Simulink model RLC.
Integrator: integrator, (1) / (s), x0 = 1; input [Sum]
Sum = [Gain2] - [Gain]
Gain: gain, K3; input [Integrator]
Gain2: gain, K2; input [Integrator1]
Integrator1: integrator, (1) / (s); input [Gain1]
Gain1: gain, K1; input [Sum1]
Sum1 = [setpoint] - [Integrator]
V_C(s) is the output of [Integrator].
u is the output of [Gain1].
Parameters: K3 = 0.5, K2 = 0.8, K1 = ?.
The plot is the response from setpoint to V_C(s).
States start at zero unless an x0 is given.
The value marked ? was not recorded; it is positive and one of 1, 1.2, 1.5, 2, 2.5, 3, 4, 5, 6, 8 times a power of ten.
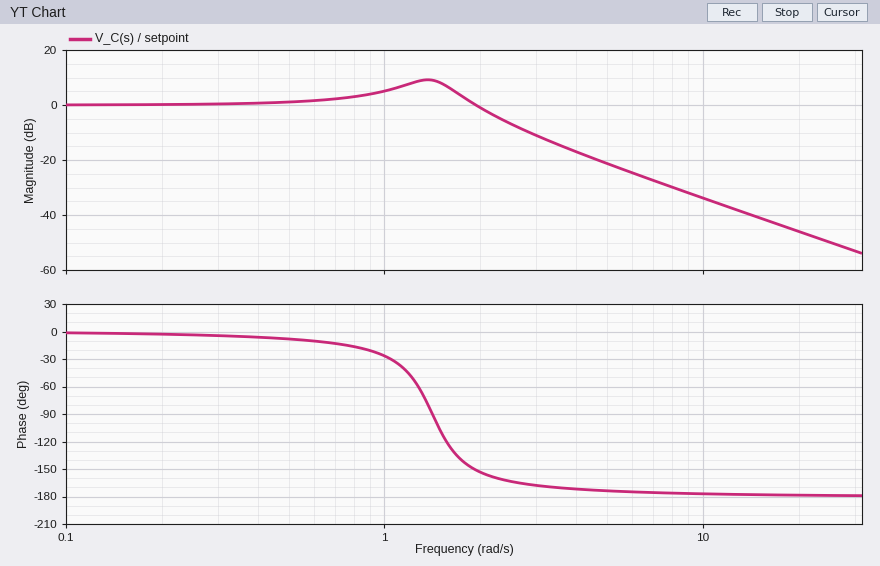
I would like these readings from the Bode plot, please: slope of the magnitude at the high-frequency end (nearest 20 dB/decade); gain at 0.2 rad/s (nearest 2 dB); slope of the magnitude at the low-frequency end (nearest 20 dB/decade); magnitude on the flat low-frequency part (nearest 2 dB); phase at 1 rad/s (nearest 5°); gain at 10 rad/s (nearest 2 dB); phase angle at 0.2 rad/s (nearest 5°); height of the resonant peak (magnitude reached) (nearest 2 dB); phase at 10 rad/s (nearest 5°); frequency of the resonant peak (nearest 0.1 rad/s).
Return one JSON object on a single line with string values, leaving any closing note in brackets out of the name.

{"slope of the magnitude at the high-frequency end": "-40 dB/decade", "gain at 0.2 rad/s": "0 dB", "slope of the magnitude at the low-frequency end": "0 dB/decade", "magnitude on the flat low-frequency part": "0 dB", "phase at 1 rad/s": "-25°", "gain at 10 rad/s": "-34 dB", "phase angle at 0.2 rad/s": "-5°", "height of the resonant peak (magnitude reached)": "10 dB", "phase at 10 rad/s": "-175°", "frequency of the resonant peak": "1.4 rad/s"}
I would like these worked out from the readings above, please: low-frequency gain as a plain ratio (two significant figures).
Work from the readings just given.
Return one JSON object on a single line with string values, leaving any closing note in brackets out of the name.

{"low-frequency gain as a plain ratio": "1.0"}
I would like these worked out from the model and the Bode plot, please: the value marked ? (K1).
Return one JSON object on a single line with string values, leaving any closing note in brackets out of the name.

{"the value marked ?": "2.5"}
